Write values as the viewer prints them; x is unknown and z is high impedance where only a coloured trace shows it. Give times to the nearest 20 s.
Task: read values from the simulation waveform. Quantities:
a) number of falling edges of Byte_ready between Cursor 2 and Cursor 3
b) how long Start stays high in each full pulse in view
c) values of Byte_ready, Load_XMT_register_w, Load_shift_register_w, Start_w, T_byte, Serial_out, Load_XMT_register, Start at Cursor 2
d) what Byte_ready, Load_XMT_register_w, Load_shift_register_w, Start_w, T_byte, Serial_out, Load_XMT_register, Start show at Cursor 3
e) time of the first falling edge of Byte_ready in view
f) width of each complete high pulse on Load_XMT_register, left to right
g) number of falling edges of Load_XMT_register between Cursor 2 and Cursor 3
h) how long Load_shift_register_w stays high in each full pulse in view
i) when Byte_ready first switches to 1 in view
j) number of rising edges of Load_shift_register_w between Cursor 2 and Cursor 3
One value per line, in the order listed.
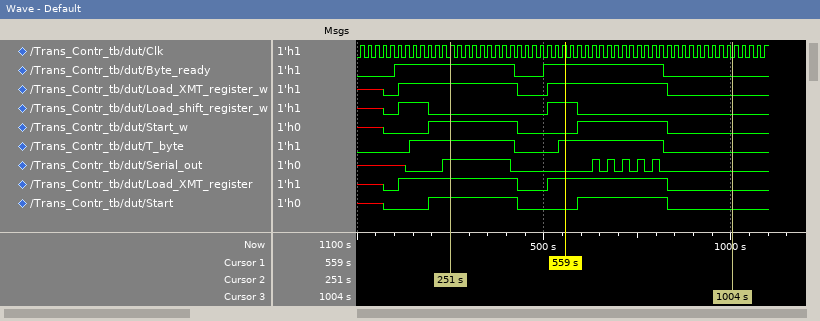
2
240 s, 240 s
Byte_ready=1, Load_XMT_register_w=1, Load_shift_register_w=0, Start_w=1, T_byte=1, Serial_out=1, Load_XMT_register=1, Start=1
Byte_ready=0, Load_XMT_register_w=0, Load_shift_register_w=0, Start_w=0, T_byte=0, Serial_out=0, Load_XMT_register=0, Start=0
420 s
320 s, 320 s
2
80 s, 80 s
100 s
1
